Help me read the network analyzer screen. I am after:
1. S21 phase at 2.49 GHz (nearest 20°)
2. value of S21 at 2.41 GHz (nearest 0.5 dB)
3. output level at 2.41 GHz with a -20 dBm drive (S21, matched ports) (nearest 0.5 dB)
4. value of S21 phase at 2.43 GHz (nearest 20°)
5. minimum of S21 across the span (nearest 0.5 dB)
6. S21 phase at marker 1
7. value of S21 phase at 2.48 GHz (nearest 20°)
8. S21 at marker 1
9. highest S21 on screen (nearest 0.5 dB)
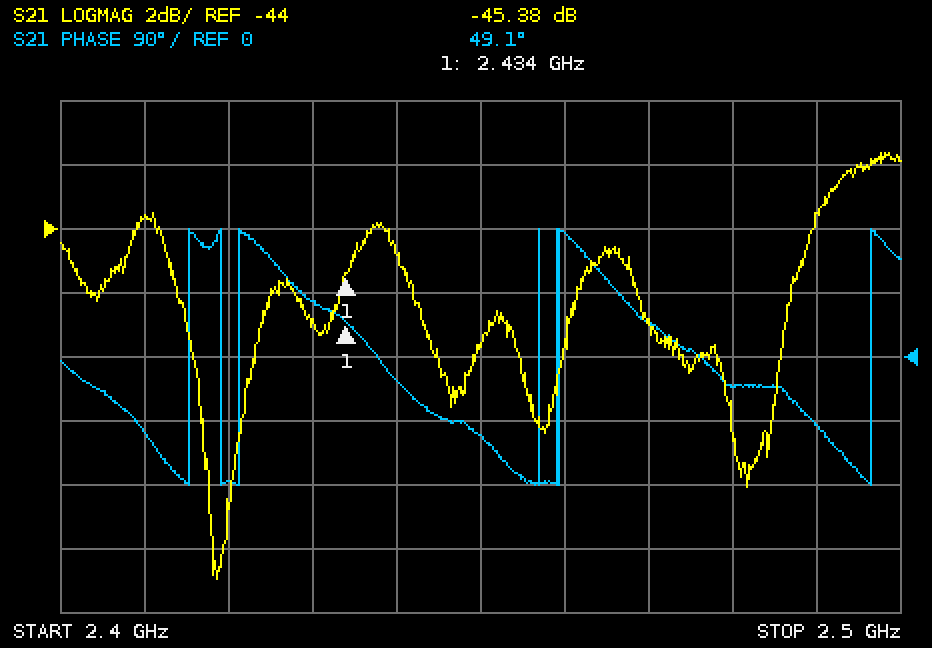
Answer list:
-100°
-43.5 dB
-63.5 dBm
80°
-55.0 dB
49.1°
-40°
-45.38 dB
-41.5 dB
